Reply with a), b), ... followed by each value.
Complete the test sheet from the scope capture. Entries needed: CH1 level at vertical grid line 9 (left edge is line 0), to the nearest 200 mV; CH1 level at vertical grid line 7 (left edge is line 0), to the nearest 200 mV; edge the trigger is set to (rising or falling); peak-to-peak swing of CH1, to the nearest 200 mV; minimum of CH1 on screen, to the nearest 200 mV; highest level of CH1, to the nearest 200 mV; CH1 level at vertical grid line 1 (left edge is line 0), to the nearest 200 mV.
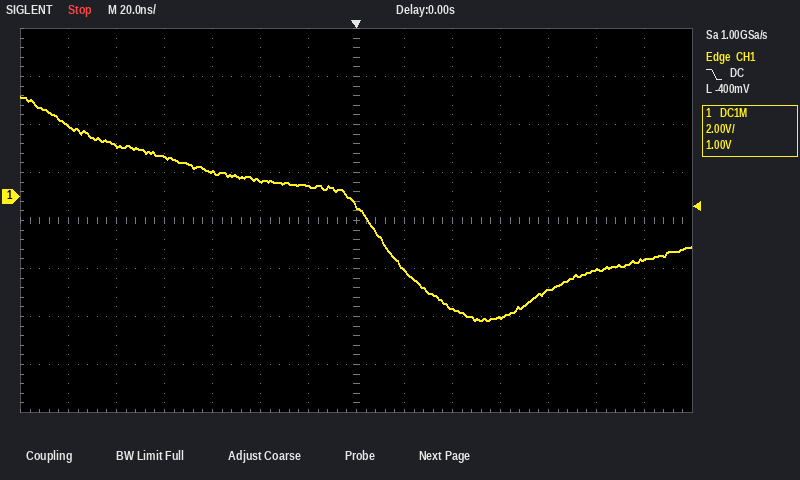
a) -4.6 V
b) -400 mV
c) falling
d) 9.4 V
e) -5.2 V
f) 4.2 V
g) 3.0 V
